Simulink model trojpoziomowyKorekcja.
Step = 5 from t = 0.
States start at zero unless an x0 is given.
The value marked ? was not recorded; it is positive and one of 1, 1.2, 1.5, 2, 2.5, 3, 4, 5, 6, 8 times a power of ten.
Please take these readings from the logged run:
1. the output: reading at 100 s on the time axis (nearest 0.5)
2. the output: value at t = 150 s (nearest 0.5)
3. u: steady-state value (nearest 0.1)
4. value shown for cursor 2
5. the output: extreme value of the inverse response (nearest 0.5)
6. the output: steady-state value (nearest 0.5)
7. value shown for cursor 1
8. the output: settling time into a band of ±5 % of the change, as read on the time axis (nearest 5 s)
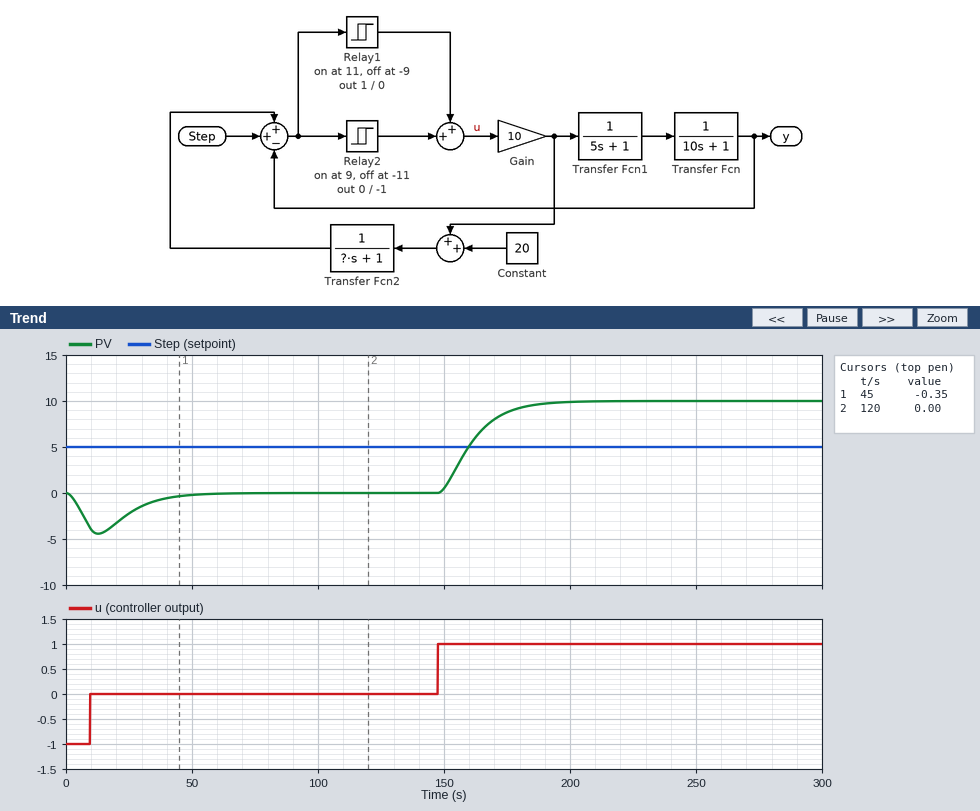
0.0
0.5
1.0
0.00
-4.5
10.0
-0.35
185 s
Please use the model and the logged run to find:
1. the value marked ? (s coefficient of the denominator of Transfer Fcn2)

400
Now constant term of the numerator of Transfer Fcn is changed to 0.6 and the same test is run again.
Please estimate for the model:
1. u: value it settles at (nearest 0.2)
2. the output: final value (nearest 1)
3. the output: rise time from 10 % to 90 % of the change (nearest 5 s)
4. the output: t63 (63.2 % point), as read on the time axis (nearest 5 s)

1.0
6
25 s
165 s
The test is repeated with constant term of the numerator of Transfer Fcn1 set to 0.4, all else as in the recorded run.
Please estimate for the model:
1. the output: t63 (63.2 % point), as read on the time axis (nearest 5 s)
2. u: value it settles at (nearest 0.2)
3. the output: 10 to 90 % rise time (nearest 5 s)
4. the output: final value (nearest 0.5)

170 s
1.0
25 s
4.0
